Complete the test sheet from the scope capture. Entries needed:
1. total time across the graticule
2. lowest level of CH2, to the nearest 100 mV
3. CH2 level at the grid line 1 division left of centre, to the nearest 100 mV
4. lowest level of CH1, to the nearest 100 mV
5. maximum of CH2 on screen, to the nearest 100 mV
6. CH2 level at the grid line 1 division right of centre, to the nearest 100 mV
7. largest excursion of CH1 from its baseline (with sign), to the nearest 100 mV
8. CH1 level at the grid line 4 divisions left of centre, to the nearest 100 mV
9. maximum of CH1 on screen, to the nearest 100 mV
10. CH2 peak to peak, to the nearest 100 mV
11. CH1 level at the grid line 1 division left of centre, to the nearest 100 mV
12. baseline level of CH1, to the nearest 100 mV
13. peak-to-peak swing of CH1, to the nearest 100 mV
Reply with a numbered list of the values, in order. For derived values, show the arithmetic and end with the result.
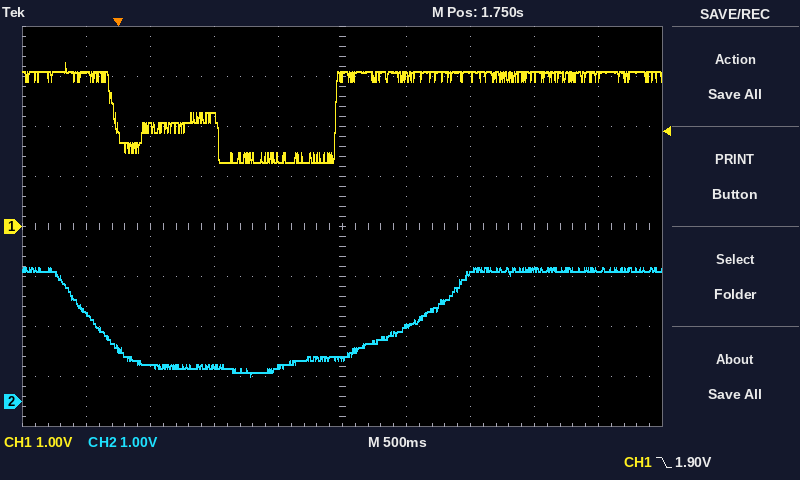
1. 5 s
2. 500 mV
3. 700 mV
4. 1.3 V
5. 2.7 V
6. 1.5 V
7. 1.3 V − (3.1 V) = -1.8 V
8. 3.1 V
9. 3.3 V
10. 2.7 V − (500 mV) = 2.2 V
11. 1.4 V
12. 3.1 V
13. 3.3 V − (1.3 V) = 2.0 V
